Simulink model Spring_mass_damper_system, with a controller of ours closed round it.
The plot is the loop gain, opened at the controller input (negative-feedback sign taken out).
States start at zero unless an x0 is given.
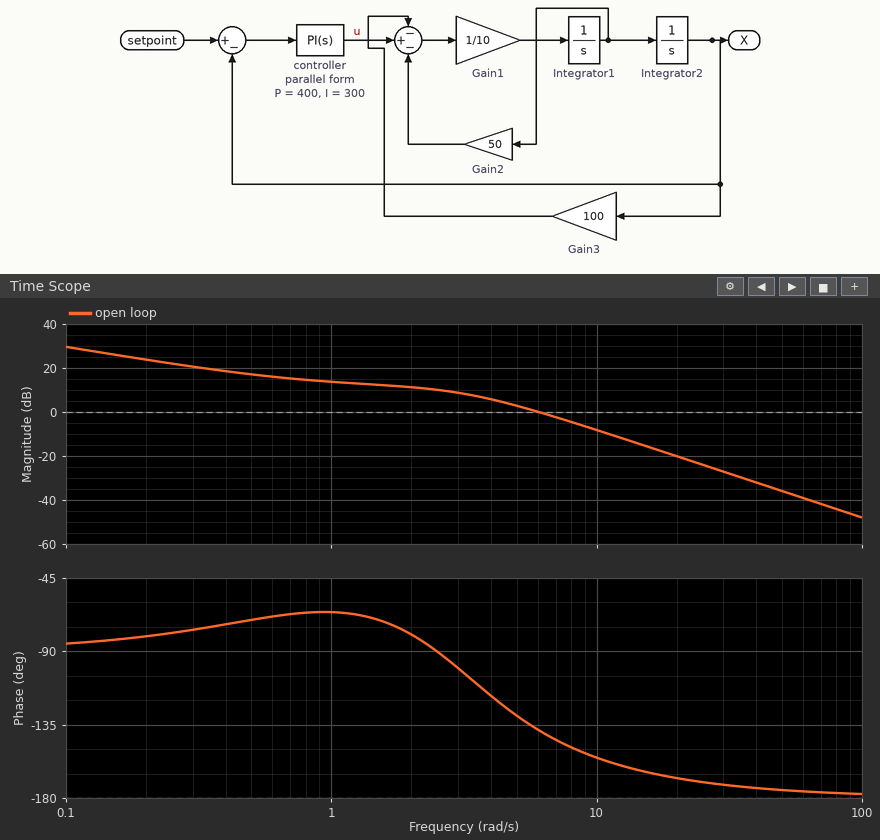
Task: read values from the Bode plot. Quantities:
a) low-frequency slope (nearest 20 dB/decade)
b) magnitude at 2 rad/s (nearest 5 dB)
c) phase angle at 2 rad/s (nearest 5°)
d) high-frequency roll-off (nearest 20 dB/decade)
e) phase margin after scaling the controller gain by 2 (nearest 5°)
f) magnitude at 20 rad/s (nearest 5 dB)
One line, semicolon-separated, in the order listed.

-20 dB/decade; 10 dB; -80°; -40 dB/decade; 30°; -20 dB
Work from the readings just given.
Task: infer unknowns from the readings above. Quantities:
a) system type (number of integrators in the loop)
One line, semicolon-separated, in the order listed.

1
